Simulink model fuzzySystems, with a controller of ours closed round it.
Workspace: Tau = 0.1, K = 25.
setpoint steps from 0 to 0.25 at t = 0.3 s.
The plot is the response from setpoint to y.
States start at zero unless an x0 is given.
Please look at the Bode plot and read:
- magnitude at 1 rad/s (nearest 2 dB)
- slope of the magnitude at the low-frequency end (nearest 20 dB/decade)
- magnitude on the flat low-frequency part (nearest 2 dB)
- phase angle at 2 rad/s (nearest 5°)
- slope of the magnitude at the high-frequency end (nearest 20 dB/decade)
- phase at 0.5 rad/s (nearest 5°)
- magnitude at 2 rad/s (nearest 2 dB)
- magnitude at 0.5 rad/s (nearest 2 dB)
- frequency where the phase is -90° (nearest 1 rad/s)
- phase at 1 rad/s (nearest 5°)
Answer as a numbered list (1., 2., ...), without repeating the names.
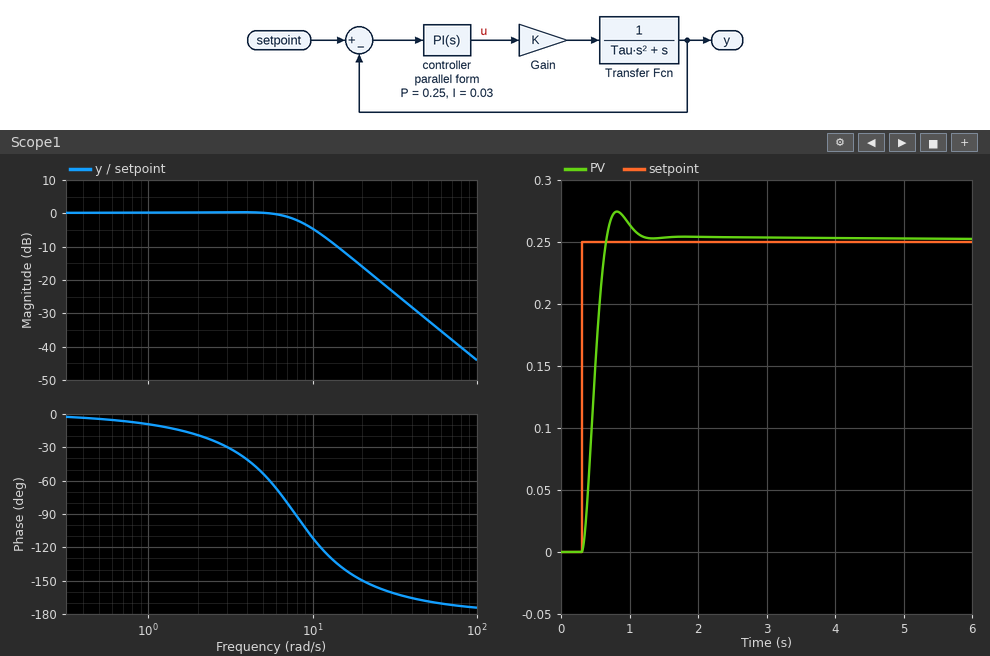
1. 0 dB
2. 0 dB/decade
3. 0 dB
4. -20°
5. -40 dB/decade
6. -5°
7. 0 dB
8. 0 dB
9. 8 rad/s
10. -10°
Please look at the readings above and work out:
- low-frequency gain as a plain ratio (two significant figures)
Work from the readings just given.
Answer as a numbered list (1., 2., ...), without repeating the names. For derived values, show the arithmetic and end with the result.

1. 10^(0 / 20) = 1.0
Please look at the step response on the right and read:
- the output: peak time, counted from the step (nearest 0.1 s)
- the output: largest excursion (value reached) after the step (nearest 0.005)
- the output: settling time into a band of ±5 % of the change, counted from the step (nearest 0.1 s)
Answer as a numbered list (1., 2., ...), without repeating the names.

1. 0.5 s
2. 0.275
3. 0.7 s
